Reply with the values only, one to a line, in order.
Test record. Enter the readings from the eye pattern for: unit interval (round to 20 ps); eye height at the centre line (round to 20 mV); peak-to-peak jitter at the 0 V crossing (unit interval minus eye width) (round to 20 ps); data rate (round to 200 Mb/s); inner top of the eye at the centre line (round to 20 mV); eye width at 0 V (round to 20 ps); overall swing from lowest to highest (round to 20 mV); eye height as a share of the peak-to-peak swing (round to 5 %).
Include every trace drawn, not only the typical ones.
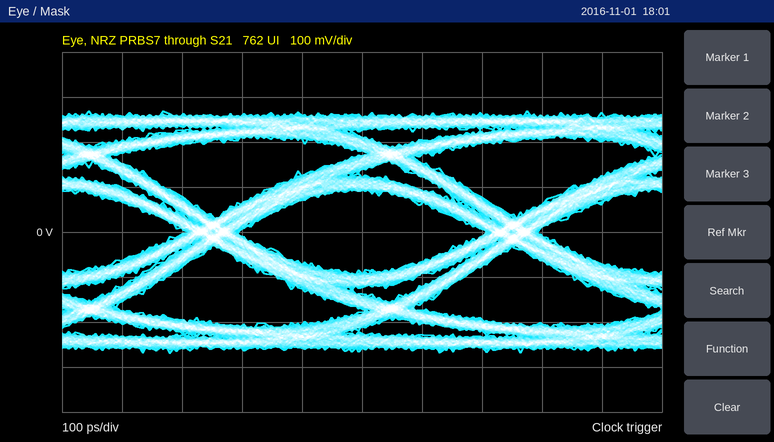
500 ps
180 mV
80 ps
2.0 Gb/s
100 mV
420 ps
540 mV
35 %
